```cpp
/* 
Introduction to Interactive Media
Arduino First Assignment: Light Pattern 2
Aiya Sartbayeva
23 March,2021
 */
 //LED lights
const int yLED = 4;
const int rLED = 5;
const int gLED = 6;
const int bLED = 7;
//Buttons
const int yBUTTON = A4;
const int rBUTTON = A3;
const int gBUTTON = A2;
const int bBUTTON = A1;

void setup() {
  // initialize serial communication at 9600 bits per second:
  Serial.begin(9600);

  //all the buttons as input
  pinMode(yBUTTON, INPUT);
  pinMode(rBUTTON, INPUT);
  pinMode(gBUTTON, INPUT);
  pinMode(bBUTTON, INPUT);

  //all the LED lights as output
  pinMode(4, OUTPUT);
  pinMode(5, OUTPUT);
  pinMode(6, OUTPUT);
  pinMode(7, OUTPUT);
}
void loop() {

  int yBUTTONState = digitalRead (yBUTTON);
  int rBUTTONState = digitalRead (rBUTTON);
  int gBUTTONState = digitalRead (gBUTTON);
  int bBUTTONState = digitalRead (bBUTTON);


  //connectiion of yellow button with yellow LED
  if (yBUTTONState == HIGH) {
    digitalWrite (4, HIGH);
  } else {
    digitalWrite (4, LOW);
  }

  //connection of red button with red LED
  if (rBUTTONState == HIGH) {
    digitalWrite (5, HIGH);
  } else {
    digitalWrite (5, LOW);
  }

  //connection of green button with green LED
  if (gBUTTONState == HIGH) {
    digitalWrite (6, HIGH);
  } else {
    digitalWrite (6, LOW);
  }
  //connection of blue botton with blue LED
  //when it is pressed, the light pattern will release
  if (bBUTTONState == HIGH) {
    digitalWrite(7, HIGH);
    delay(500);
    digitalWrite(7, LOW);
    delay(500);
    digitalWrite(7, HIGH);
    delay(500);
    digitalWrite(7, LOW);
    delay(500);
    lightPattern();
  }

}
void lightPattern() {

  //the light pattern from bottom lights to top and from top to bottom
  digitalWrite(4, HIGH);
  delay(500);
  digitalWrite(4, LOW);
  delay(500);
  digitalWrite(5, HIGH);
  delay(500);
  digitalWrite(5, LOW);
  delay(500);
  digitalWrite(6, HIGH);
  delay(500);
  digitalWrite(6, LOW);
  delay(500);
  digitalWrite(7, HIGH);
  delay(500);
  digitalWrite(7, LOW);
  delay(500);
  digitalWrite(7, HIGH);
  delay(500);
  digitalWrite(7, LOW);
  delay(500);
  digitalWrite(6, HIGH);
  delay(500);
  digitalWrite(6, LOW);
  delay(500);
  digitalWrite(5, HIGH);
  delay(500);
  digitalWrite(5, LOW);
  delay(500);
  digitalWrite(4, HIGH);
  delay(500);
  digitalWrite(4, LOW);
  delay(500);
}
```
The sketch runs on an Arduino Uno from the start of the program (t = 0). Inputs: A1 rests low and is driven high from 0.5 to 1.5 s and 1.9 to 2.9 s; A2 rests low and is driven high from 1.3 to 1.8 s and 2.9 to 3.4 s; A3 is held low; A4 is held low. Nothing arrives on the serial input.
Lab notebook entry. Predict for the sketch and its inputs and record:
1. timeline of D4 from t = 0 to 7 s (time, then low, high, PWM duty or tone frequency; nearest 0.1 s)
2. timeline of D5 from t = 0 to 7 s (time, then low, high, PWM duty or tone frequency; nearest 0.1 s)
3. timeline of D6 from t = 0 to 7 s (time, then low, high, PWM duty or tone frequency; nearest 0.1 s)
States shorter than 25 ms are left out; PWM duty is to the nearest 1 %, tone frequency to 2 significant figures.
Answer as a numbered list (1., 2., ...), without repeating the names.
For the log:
1. 0 s low; 2.5 s high; 3 s low
2. 0 s low; 3.5 s high; 4 s low
3. 0 s low; 4.5 s high; 5 s low
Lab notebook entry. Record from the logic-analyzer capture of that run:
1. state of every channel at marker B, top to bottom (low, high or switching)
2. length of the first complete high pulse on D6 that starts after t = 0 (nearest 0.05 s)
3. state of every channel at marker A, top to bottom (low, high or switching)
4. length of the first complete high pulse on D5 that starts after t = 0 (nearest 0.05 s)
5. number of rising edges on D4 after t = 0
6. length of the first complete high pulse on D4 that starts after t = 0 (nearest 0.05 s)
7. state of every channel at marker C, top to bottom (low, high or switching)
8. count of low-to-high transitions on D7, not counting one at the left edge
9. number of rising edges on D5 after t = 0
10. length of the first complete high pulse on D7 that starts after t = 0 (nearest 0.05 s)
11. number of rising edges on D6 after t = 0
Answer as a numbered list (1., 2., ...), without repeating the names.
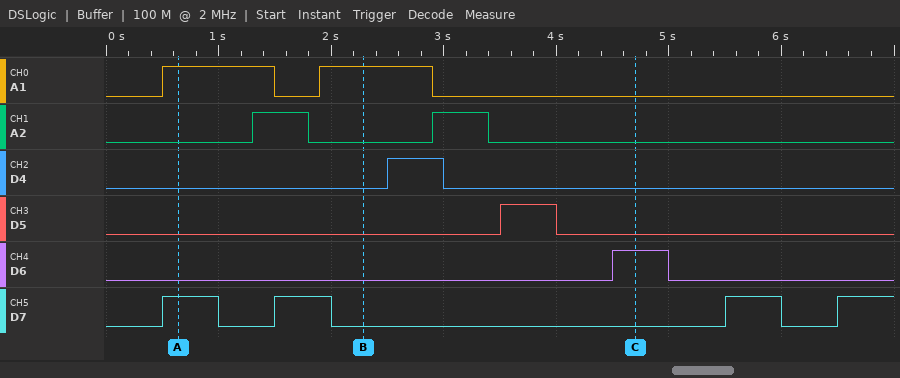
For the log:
1. A1 high, A2 low, D4 low, D5 low, D6 low, D7 low
2. 0.50 s
3. A1 high, A2 low, D4 low, D5 low, D6 low, D7 high
4. 0.50 s
5. 1
6. 0.50 s
7. A1 low, A2 low, D4 low, D5 low, D6 high, D7 low
8. 4
9. 1
10. 0.50 s
11. 1
